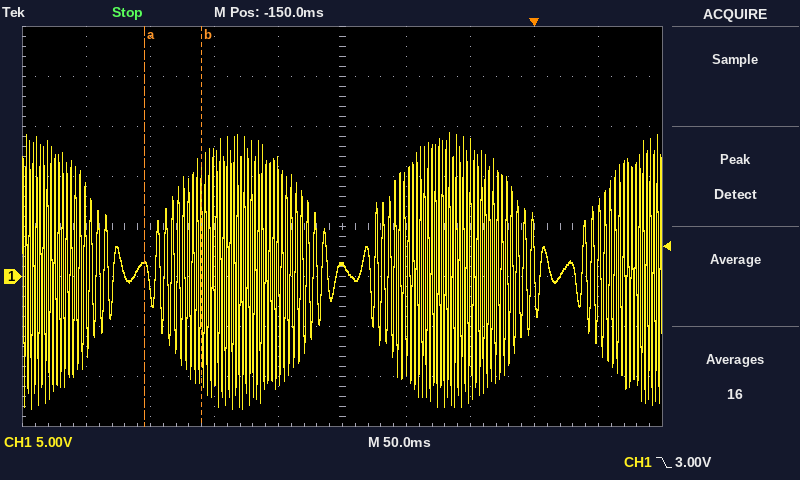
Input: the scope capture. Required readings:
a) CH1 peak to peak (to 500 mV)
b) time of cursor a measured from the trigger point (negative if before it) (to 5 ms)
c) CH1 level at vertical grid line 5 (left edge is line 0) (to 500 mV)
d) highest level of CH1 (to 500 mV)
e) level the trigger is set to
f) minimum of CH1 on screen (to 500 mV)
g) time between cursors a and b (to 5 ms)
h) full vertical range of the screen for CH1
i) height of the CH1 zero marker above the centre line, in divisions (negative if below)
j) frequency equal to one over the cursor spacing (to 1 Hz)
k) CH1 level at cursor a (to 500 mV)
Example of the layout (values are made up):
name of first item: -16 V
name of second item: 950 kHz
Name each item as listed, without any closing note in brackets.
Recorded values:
CH1 peak to peak: 27.5 V
time of cursor a measured from the trigger point (negative if before it): -305 ms
CH1 level at vertical grid line 5 (left edge is line 0): 1.0 V
highest level of CH1: 14.5 V
level the trigger is set to: 3.00 V
minimum of CH1 on screen: -13.0 V
time between cursors a and b: 45 ms
full vertical range of the screen for CH1: 40 V
height of the CH1 zero marker above the centre line, in divisions: -1.0 div
frequency equal to one over the cursor spacing: 22 Hz
CH1 level at cursor a: 1.0 V
